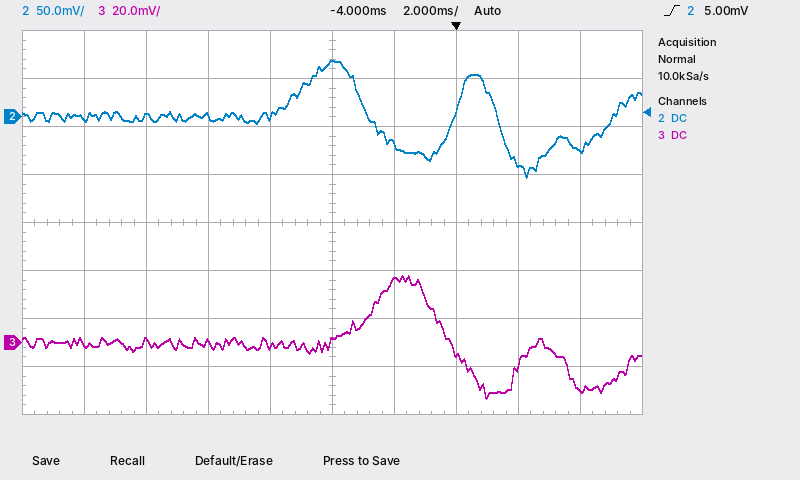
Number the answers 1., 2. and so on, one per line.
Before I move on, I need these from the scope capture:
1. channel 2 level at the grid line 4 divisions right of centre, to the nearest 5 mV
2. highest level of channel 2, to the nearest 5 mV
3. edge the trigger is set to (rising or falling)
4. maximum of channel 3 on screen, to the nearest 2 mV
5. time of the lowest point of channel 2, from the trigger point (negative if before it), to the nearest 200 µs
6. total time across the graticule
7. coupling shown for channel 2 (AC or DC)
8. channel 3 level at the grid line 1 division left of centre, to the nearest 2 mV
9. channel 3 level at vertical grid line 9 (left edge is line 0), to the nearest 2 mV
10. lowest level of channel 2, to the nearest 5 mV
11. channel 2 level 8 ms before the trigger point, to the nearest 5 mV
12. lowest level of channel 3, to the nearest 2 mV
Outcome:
1. -35 mV
2. 60 mV
3. rising
4. 28 mV
5. +2.2 ms
6. 20 ms
7. DC
8. -2 mV
9. -20 mV
10. -65 mV
11. 0 mV
12. -24 mV
